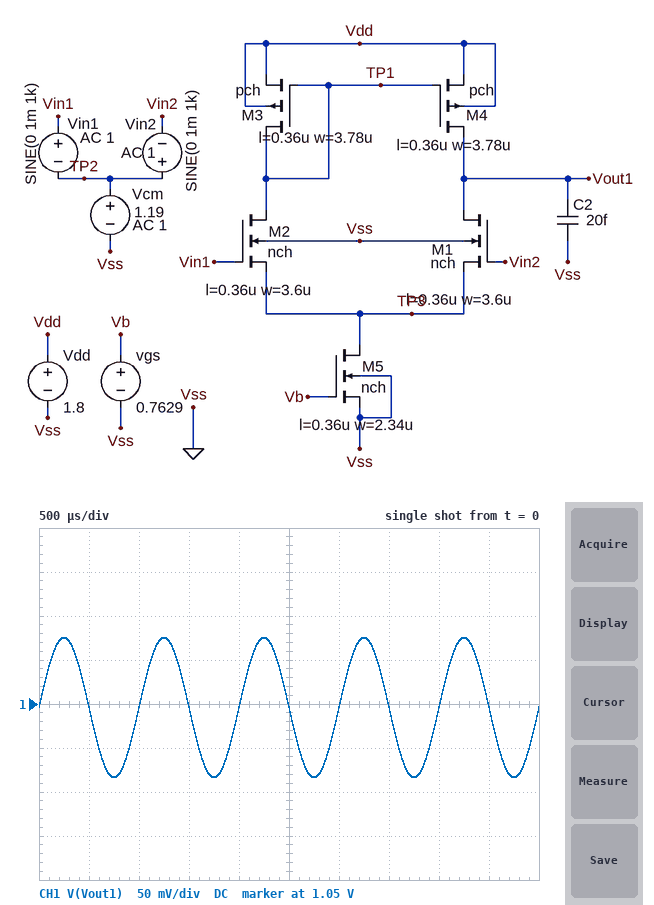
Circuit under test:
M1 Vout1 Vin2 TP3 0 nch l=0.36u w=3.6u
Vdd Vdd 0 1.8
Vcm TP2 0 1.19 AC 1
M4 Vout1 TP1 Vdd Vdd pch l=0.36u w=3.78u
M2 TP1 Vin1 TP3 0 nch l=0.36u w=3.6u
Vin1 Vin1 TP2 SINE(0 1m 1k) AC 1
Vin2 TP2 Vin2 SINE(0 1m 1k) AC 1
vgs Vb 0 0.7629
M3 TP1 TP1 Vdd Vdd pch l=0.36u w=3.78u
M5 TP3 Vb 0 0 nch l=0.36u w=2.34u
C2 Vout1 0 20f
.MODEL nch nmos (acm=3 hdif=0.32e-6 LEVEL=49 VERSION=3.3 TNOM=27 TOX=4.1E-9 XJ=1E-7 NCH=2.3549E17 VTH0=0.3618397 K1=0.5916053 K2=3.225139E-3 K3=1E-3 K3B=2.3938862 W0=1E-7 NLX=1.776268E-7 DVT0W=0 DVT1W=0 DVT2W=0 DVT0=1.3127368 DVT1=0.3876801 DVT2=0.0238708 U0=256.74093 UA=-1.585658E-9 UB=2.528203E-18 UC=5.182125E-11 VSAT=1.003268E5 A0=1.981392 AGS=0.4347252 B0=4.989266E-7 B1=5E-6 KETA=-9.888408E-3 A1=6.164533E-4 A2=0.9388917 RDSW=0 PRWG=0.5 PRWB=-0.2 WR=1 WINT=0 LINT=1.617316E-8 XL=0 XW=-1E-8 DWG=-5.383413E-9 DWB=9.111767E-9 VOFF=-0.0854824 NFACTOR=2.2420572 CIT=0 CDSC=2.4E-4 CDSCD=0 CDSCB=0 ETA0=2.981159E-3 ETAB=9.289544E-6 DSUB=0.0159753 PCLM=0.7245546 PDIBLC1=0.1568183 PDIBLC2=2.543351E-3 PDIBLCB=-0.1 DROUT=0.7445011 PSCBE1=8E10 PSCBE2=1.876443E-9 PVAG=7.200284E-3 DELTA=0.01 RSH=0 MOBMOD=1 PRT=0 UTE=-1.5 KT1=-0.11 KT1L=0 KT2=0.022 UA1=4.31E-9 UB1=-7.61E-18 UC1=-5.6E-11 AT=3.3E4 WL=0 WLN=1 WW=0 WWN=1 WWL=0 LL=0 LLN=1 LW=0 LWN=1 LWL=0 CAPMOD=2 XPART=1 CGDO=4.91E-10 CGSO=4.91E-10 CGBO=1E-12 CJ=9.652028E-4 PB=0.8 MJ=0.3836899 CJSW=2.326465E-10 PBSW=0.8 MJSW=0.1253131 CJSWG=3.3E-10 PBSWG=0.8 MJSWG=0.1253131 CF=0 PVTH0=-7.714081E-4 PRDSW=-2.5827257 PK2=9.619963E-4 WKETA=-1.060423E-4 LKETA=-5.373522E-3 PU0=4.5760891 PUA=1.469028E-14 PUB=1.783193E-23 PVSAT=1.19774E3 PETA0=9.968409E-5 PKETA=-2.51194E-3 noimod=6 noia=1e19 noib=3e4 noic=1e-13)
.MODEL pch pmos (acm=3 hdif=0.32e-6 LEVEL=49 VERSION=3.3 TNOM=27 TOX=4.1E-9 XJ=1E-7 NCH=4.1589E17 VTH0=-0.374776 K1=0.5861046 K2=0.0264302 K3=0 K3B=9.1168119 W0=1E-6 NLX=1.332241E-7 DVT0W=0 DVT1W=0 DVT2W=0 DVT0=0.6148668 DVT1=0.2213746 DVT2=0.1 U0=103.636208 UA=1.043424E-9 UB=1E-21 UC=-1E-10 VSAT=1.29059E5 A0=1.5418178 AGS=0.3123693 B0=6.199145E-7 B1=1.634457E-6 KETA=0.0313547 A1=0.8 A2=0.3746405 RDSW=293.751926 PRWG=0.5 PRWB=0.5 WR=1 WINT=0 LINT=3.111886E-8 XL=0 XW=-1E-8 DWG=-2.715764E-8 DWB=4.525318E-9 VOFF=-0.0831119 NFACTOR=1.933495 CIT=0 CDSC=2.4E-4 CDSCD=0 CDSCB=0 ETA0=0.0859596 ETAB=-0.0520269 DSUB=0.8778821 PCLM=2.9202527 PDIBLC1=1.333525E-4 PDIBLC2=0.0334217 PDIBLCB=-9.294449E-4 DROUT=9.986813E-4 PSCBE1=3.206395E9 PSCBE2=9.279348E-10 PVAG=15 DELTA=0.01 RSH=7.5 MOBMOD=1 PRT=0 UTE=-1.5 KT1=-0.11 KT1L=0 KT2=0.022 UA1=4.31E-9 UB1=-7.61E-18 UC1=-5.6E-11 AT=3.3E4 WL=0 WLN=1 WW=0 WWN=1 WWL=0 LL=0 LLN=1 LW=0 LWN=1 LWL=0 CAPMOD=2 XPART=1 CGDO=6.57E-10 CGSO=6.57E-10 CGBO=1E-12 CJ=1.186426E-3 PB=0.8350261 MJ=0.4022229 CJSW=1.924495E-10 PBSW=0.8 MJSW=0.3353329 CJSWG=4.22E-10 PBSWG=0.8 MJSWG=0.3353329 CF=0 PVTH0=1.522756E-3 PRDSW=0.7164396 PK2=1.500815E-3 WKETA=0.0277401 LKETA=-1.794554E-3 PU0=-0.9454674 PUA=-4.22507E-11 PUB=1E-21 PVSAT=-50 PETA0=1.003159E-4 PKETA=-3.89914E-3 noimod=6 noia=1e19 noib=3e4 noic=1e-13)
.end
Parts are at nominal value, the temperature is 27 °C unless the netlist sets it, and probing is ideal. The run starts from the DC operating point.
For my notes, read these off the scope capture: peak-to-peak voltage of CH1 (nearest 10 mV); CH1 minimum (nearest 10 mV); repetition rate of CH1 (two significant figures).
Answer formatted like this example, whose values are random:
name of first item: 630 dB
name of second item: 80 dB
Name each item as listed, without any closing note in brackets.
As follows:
peak-to-peak voltage of CH1: 160 mV
CH1 minimum: 970 mV
repetition rate of CH1: 1.0 kHz
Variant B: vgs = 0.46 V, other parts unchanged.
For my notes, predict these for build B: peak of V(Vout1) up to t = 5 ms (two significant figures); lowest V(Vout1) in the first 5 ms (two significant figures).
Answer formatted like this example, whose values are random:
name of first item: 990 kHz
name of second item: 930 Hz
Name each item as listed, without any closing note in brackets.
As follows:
peak of V(Vout1) up to t = 5 ms: 1.4 V
lowest V(Vout1) in the first 5 ms: 1.3 V
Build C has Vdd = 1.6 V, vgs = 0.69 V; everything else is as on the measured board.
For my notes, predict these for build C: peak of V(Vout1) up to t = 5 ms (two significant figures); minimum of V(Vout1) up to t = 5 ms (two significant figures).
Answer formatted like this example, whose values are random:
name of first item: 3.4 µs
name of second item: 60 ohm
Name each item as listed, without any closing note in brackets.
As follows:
peak of V(Vout1) up to t = 5 ms: 1.0 V
minimum of V(Vout1) up to t = 5 ms: 840 mV
